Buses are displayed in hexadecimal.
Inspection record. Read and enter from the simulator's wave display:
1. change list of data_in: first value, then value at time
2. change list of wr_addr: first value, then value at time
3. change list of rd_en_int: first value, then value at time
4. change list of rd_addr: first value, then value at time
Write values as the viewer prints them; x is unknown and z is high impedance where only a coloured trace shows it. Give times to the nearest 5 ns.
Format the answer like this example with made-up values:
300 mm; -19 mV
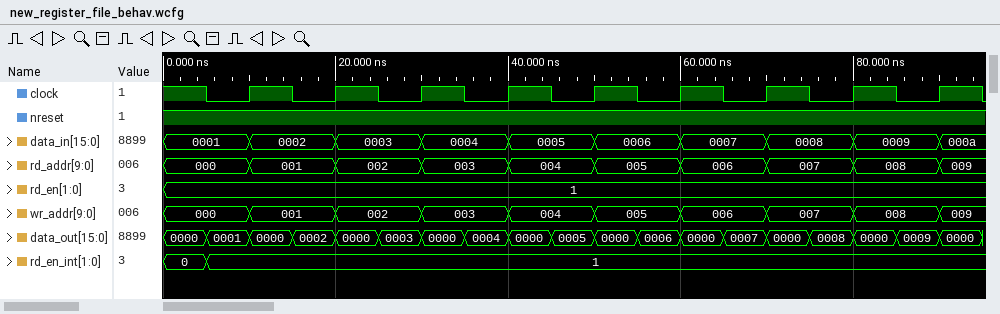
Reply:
0001, 0002 at 10 ns, 0003 at 20 ns, 0004 at 30 ns, 0005 at 40 ns, 0006 at 50 ns, 0007 at 60 ns, 0008 at 70 ns, 0009 at 80 ns, 000a at 90 ns; 000, 001 at 10 ns, 002 at 20 ns, 003 at 30 ns, 004 at 40 ns, 005 at 50 ns, 006 at 60 ns, 007 at 70 ns, 008 at 80 ns, 009 at 90 ns; 0, 1 at 5 ns; 000, 001 at 10 ns, 002 at 20 ns, 003 at 30 ns, 004 at 40 ns, 005 at 50 ns, 006 at 60 ns, 007 at 70 ns, 008 at 80 ns, 009 at 90 ns
